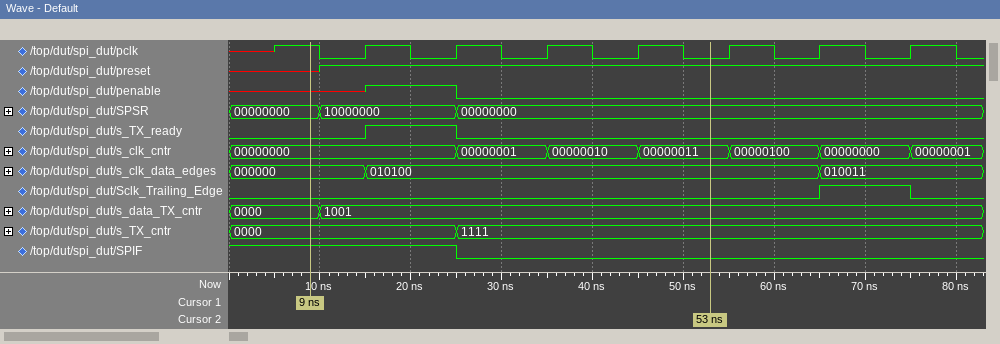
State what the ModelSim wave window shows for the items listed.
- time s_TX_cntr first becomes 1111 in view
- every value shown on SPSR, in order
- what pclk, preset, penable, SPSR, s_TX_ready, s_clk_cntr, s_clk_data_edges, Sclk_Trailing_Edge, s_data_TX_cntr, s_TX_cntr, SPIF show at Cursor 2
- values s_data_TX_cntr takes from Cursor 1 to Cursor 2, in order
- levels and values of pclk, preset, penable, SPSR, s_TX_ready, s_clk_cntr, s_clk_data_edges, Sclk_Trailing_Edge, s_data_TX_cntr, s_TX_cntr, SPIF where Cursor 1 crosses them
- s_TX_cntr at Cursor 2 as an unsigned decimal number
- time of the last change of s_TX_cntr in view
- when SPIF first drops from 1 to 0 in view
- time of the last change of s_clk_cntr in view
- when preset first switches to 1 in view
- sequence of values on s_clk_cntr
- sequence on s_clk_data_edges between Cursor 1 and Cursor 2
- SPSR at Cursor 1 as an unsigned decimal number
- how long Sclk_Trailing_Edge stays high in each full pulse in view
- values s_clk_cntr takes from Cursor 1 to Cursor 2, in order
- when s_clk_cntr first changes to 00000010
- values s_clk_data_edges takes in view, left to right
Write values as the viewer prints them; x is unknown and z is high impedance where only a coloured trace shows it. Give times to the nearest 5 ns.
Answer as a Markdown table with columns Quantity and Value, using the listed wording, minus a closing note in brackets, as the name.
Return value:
| Quantity | Value |
|---|---|
| time s_TX_cntr first becomes 1111 in view | 25 ns |
| every value shown on SPSR, in order | 00000000, 10000000, 00000000 |
| what pclk, preset, penable, SPSR, s_TX_ready, s_clk_cntr, s_clk_data_edges, Sclk_Trailing_Edge, s_data_TX_cntr, s_TX_cntr, SPIF show at Cursor 2 | pclk=0, preset=1, penable=0, SPSR=00000000, s_TX_ready=0, s_clk_cntr=00000011, s_clk_data_edges=010100, Sclk_Trailing_Edge=0, s_data_TX_cntr=1001, s_TX_cntr=1111, SPIF=0 |
| values s_data_TX_cntr takes from Cursor 1 to Cursor 2, in order | 0000, 1001 |
| levels and values of pclk, preset, penable, SPSR, s_TX_ready, s_clk_cntr, s_clk_data_edges, Sclk_Trailing_Edge, s_data_TX_cntr, s_TX_cntr, SPIF where Cursor 1 crosses them | pclk=1, preset=x, penable=x, SPSR=00000000, s_TX_ready=0, s_clk_cntr=00000000, s_clk_data_edges=000000, Sclk_Trailing_Edge=0, s_data_TX_cntr=0000, s_TX_cntr=0000, SPIF=1 |
| s_TX_cntr at Cursor 2 as an unsigned decimal number | 15 |
| time of the last change of s_TX_cntr in view | 25 ns |
| when SPIF first drops from 1 to 0 in view | 25 ns |
| time of the last change of s_clk_cntr in view | 75 ns |
| when preset first switches to 1 in view | 10 ns |
| sequence of values on s_clk_cntr | 00000000, 00000001, 00000010, 00000011, 00000100, 00000000, 00000001 |
| sequence on s_clk_data_edges between Cursor 1 and Cursor 2 | 000000, 010100 |
| SPSR at Cursor 1 as an unsigned decimal number | 0 |
| how long Sclk_Trailing_Edge stays high in each full pulse in view | 10 ns |
| values s_clk_cntr takes from Cursor 1 to Cursor 2, in order | 00000000, 00000001, 00000010, 00000011 |
| when s_clk_cntr first changes to 00000010 | 35 ns |
| values s_clk_data_edges takes in view, left to right | 000000, 010100, 010011 |
